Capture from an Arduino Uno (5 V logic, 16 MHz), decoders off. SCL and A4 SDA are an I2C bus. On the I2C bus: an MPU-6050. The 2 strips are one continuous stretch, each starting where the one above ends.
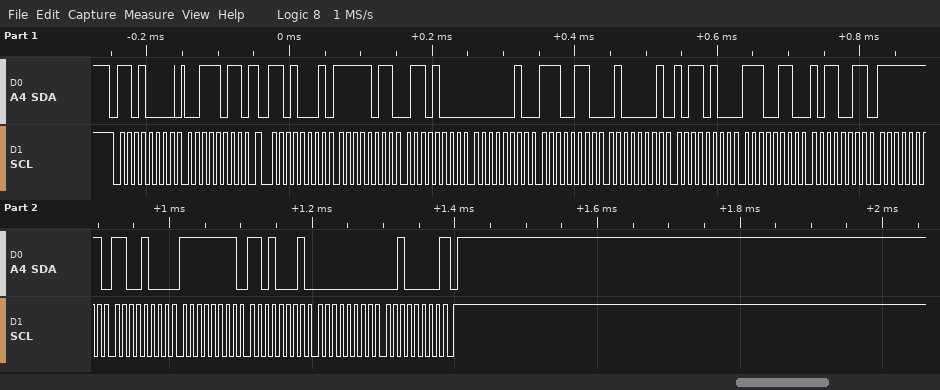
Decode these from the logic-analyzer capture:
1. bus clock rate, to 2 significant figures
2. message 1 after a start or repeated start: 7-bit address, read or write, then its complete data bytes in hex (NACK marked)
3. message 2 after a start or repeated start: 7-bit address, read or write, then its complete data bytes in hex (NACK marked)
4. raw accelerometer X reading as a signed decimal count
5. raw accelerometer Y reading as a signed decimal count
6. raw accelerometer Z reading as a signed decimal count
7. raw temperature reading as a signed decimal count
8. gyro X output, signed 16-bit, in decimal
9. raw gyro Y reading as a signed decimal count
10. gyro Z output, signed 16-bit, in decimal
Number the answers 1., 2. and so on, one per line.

1. 100 kHz
2. 0x68 write: 3B
3. 0x68 read: FB 68 02 E6 41 B4 E6 B3 FF C8 FF D1 00 20 NACK
4. -1176
5. 742
6. 16820
7. -6477
8. -56
9. -47
10. 32
